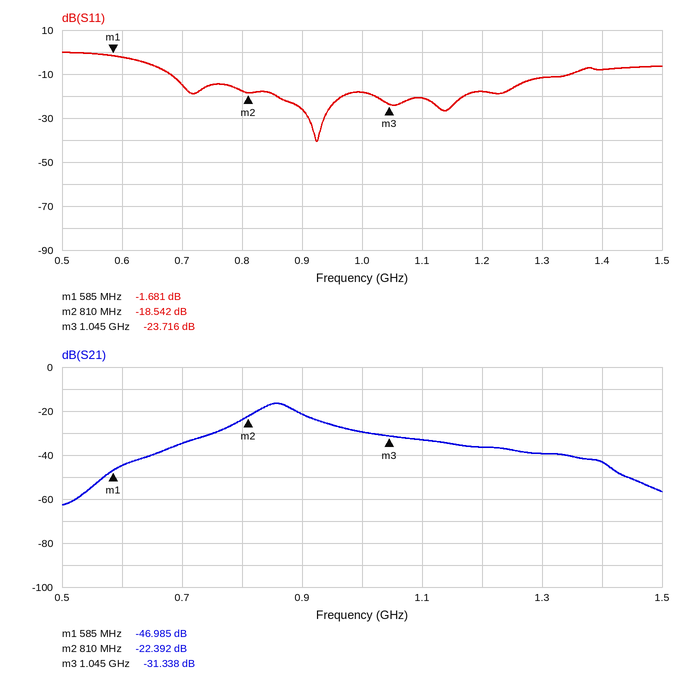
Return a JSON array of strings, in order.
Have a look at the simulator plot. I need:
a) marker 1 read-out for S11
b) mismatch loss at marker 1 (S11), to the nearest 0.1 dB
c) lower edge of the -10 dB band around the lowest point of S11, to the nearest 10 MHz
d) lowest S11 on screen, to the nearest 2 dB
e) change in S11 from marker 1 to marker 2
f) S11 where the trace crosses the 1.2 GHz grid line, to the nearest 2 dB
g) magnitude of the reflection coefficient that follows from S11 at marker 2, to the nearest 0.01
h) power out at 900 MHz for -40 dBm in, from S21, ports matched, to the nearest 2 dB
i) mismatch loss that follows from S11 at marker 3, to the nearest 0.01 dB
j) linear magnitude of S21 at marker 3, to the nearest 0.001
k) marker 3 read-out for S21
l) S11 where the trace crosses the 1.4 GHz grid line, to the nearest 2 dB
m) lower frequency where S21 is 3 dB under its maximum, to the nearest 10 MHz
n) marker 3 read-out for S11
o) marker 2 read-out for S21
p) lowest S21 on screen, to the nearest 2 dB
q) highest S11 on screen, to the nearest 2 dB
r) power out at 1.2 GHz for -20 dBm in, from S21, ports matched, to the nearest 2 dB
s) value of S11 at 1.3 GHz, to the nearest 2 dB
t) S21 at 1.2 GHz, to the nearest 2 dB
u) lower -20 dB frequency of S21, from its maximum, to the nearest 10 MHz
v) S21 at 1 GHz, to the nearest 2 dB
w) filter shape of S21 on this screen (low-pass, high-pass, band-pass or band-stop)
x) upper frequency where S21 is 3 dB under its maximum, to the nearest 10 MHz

["-1.681 dB", "4.9 dB", "680 MHz", "-40 dB", "-16.861 dB", "-18 dB", "0.12", "-62 dBm", "0.02 dB", "0.027", "-31.338 dB", "-8 dB", "830 MHz", "-23.716 dB", "-22.392 dB", "-62 dB", "0 dB", "-56 dBm", "-12 dB", "-36 dB", "680 MHz", "-30 dB", "band-pass", "890 MHz"]
